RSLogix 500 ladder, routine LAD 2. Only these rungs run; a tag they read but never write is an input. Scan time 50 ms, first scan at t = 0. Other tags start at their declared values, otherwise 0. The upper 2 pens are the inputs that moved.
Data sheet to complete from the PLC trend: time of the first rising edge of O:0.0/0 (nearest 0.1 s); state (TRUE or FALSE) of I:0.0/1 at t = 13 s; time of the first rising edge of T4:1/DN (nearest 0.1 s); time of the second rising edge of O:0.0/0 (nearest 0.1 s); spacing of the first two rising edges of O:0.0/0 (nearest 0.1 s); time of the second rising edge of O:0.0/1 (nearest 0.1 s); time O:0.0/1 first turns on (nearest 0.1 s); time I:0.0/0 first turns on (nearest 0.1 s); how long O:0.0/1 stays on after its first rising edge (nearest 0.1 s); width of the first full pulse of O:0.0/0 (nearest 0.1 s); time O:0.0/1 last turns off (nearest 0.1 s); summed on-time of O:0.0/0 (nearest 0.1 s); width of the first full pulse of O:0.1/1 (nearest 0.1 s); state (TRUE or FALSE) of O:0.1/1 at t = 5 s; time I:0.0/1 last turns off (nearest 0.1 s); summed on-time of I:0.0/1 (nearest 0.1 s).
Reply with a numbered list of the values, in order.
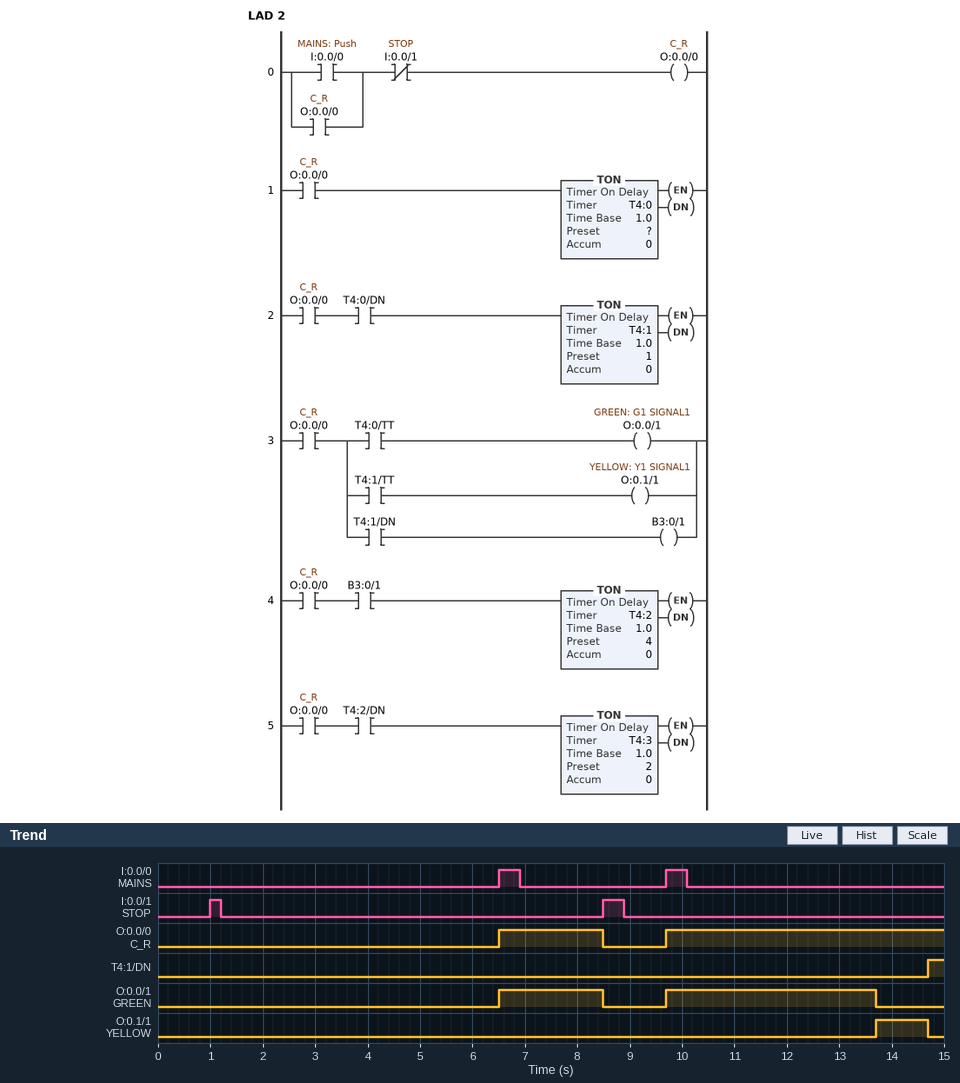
1. 6.5 s
2. FALSE
3. 14.7 s
4. 9.7 s
5. 3.2 s
6. 9.7 s
7. 6.5 s
8. 6.5 s
9. 2.0 s
10. 2.0 s
11. 13.7 s
12. 7.3 s
13. 1.0 s
14. FALSE
15. 8.9 s
16. 0.6 s
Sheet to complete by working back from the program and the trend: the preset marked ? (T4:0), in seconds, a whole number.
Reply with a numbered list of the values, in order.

1. 4 s
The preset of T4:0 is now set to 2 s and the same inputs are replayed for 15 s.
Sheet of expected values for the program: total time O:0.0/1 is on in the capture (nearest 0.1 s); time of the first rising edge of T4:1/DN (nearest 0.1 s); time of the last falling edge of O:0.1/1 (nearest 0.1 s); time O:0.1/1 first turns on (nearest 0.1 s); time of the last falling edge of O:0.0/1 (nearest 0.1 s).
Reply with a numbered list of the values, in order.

1. 4.0 s
2. 12.7 s
3. 12.7 s
4. 11.7 s
5. 11.7 s
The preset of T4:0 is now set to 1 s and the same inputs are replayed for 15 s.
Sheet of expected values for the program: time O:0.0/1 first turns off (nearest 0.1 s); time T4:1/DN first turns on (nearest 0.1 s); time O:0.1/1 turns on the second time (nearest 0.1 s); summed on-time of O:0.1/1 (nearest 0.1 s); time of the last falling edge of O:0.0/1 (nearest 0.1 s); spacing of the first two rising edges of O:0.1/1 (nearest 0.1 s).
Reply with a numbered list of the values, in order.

1. 7.5 s
2. 11.7 s
3. 10.7 s
4. 2.0 s
5. 10.7 s
6. 3.2 s
